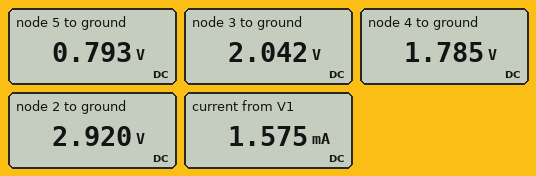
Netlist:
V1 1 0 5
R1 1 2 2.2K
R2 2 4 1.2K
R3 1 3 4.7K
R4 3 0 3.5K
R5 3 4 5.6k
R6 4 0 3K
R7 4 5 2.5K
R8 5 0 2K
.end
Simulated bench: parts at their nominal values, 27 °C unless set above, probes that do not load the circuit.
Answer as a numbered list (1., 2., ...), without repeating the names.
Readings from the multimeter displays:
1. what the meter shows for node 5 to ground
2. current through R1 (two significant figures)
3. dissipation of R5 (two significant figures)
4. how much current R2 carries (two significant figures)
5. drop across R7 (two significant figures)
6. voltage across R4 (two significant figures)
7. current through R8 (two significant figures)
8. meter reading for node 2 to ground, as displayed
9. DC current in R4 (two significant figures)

1. 0.793 V
2. 950 µA
3. 12 µW
4. 950 µA
5. 990 mV
6. 2.0 V
7. 400 µA
8. 2.920 V
9. 580 µA
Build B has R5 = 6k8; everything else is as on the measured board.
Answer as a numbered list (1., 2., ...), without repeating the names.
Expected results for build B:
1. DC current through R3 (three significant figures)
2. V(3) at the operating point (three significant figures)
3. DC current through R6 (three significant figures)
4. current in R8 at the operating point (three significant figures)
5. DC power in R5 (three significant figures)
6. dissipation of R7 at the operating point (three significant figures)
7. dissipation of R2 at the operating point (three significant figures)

1. 627 µA
2. 2.05 V
3. 593 µA
4. 395 µA
5. 11.1 µW
6. 390 µW
7. 1.08 mW
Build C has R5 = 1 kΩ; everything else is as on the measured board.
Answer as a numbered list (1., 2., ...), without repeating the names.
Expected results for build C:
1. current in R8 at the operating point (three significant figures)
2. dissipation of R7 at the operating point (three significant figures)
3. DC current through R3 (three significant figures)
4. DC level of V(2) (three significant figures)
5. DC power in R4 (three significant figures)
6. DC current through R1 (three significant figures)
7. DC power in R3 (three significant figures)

1. 410 µA
2. 420 µW
3. 651 µA
4. 2.96 V
5. 1.08 mW
6. 928 µA
7. 1.99 mW
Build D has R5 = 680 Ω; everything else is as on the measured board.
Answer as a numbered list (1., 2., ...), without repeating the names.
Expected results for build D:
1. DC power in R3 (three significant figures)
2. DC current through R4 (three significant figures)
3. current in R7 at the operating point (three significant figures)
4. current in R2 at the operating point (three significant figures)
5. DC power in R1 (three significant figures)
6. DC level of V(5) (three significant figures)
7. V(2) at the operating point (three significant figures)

1. 2.01 mW
2. 550 µA
3. 412 µA
4. 925 µA
5. 1.88 mW
6. 824 mV
7. 2.96 V
